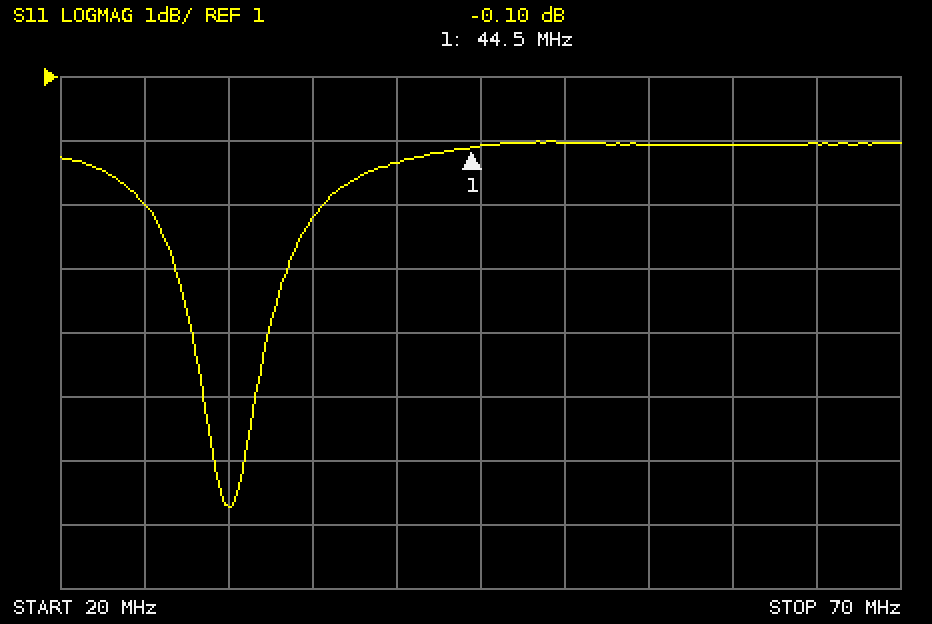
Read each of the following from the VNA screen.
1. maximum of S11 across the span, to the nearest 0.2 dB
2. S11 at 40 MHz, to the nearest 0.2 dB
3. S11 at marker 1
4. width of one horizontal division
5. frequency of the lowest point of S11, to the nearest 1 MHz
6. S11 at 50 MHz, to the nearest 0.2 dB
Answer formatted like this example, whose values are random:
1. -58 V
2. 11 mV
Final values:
1. 0.0 dB
2. -0.4 dB
3. -0.10 dB
4. 5 MHz
5. 30 MHz
6. 0.0 dB
